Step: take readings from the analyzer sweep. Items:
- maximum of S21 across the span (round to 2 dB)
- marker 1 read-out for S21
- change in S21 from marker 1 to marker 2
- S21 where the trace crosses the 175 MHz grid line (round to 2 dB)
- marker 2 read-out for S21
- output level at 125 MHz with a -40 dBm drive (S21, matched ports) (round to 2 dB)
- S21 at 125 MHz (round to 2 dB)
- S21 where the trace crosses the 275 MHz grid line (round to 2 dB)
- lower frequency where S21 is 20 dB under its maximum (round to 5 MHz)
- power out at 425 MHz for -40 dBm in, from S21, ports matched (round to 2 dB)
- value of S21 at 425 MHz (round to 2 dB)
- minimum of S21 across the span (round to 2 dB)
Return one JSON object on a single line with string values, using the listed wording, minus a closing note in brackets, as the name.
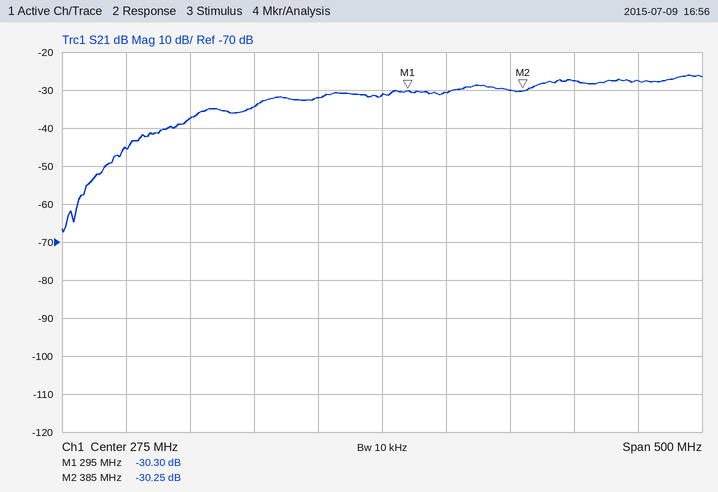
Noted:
{"maximum of S21 across the span": "-26 dB", "marker 1 read-out for S21": "-30.30 dB", "change in S21 from marker 1 to marker 2": "0.05 dB", "S21 where the trace crosses the 175 MHz grid line": "-34 dB", "marker 2 read-out for S21": "-30.25 dB", "output level at 125 MHz with a -40 dBm drive (S21, matched ports)": "-78 dBm", "S21 at 125 MHz": "-38 dB", "S21 where the trace crosses the 275 MHz grid line": "-32 dB", "lower frequency where S21 is 20 dB under its maximum": "70 MHz", "power out at 425 MHz for -40 dBm in, from S21, ports matched": "-68 dBm", "value of S21 at 425 MHz": "-28 dB", "minimum of S21 across the span": "-68 dB"}
